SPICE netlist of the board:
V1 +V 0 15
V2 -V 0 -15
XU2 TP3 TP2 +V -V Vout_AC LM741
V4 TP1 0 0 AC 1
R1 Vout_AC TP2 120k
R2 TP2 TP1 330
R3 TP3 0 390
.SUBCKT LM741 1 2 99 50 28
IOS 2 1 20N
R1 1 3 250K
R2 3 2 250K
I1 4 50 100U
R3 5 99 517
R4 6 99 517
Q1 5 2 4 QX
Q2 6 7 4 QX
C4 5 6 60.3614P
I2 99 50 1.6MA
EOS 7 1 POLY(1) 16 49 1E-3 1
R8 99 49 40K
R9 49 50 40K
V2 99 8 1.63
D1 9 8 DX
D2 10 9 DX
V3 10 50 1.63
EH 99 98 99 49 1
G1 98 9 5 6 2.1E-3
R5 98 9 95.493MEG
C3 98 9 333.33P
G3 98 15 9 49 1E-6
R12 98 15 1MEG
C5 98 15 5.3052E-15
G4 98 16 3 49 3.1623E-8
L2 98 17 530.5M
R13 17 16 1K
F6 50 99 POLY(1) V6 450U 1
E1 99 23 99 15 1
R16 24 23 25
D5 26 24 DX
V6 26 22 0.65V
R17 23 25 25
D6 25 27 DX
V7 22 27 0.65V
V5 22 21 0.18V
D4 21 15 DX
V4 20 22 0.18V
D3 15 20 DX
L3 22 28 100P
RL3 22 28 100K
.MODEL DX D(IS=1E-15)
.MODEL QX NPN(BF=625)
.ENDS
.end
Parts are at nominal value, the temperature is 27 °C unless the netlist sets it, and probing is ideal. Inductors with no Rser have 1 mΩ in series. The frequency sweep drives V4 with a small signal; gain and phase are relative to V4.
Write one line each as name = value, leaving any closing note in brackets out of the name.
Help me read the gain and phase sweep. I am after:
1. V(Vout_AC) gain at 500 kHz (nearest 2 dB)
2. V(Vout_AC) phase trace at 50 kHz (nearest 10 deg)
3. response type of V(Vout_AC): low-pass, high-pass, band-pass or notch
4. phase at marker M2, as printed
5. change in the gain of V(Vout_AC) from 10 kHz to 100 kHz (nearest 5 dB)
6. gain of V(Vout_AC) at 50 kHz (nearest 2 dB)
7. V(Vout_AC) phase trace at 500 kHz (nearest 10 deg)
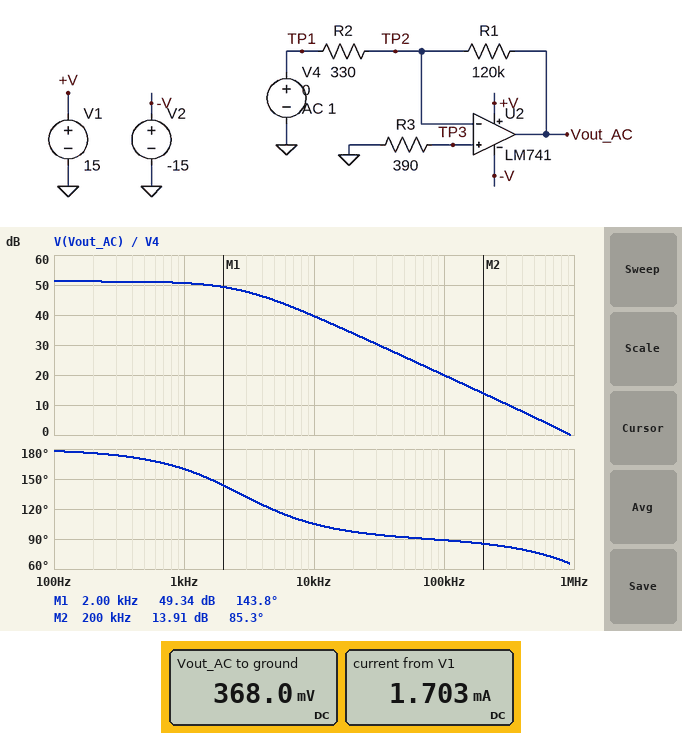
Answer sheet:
V(Vout_AC) gain at 500 kHz = 6 dB
V(Vout_AC) phase trace at 50 kHz = 90 deg
response type of V(Vout_AC): low-pass, high-pass, band-pass or notch = low-pass
phase at marker M2, as printed = 85.3 deg
change in the gain of V(Vout_AC) from 10 kHz to 100 kHz = -20 dB
gain of V(Vout_AC) at 50 kHz = 26 dB
V(Vout_AC) phase trace at 500 kHz = 80 deg
